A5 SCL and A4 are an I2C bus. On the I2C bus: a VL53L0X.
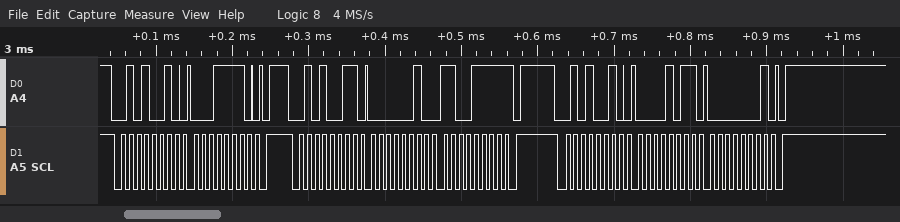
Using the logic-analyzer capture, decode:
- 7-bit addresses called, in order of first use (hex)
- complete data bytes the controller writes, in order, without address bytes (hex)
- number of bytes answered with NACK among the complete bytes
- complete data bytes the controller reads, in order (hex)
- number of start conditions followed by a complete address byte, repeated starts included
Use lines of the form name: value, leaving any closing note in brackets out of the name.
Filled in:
7-bit addresses called, in order of first use: 0x29
complete data bytes the controller writes, in order, without address bytes: 1E 0B 01
number of bytes answered with NACK among the complete bytes: 1
complete data bytes the controller reads, in order: 02 CF
number of start conditions followed by a complete address byte, repeated starts included: 3
